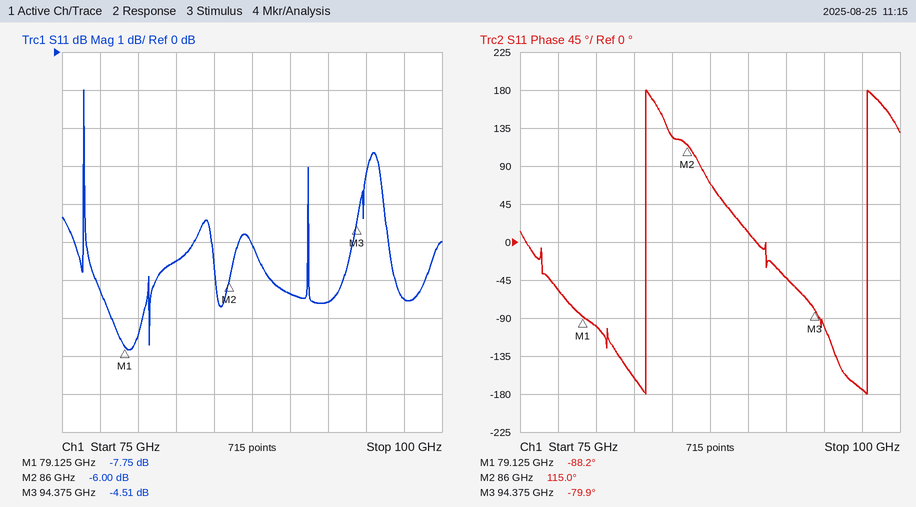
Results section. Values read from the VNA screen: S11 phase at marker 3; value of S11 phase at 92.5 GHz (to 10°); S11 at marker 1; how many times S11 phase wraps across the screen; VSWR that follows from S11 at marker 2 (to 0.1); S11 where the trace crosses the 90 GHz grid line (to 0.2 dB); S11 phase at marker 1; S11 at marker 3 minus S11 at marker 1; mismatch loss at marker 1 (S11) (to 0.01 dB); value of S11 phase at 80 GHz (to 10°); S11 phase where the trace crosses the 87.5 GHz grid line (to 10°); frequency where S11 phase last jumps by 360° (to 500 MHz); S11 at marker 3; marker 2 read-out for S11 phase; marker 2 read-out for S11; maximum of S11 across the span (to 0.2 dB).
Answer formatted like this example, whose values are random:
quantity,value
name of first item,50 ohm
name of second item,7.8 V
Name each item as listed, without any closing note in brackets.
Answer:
quantity,value
S11 phase at marker 3,-79.9°
value of S11 phase at 92.5 GHz,-40°
S11 at marker 1,-7.75 dB
how many times S11 phase wraps across the screen,2
VSWR that follows from S11 at marker 2,3.0
S11 where the trace crosses the 90 GHz grid line,-6.4 dB
S11 phase at marker 1,-88.2°
S11 at marker 3 minus S11 at marker 1,3.24 dB
mismatch loss at marker 1 (S11),0.80 dB
value of S11 phase at 80 GHz,-100°
S11 phase where the trace crosses the 87.5 GHz grid line,70°
frequency where S11 phase last jumps by 360°,98.0 GHz
S11 at marker 3,-4.51 dB
marker 2 read-out for S11 phase,115.0°
marker 2 read-out for S11,-6.00 dB
maximum of S11 across the span,-1.0 dB
